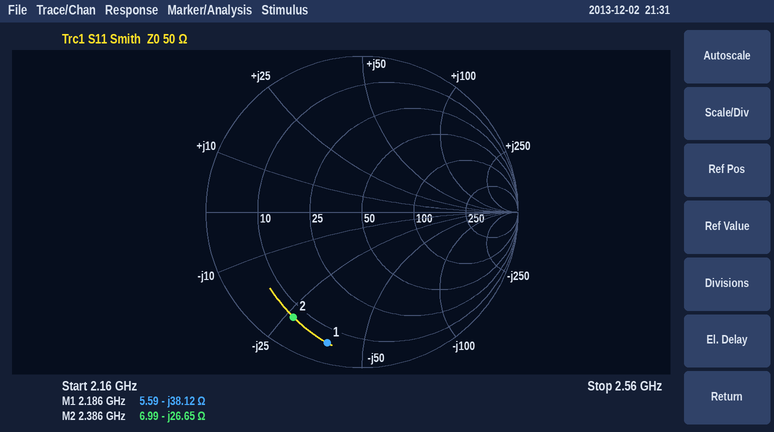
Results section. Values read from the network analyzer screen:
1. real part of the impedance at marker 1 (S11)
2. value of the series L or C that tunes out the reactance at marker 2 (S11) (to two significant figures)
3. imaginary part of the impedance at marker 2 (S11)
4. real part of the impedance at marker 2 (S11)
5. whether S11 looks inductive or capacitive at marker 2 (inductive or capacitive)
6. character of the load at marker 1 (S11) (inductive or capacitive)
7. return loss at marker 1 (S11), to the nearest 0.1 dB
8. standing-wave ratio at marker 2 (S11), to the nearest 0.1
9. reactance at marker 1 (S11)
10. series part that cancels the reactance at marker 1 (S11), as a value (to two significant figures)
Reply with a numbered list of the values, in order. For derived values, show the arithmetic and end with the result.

1. 5.59 Ω
2. L = 26.65 Ω/(2π × 2.386 GHz) ≈ 1.8 nH
3. -26.65 Ω
4. 6.99 Ω
5. capacitive
6. capacitive
7. 1.2 dB
8. 9.2
9. -38.12 Ω
10. L = 38.12 Ω/(2π × 2.186 GHz) ≈ 2.8 nH
